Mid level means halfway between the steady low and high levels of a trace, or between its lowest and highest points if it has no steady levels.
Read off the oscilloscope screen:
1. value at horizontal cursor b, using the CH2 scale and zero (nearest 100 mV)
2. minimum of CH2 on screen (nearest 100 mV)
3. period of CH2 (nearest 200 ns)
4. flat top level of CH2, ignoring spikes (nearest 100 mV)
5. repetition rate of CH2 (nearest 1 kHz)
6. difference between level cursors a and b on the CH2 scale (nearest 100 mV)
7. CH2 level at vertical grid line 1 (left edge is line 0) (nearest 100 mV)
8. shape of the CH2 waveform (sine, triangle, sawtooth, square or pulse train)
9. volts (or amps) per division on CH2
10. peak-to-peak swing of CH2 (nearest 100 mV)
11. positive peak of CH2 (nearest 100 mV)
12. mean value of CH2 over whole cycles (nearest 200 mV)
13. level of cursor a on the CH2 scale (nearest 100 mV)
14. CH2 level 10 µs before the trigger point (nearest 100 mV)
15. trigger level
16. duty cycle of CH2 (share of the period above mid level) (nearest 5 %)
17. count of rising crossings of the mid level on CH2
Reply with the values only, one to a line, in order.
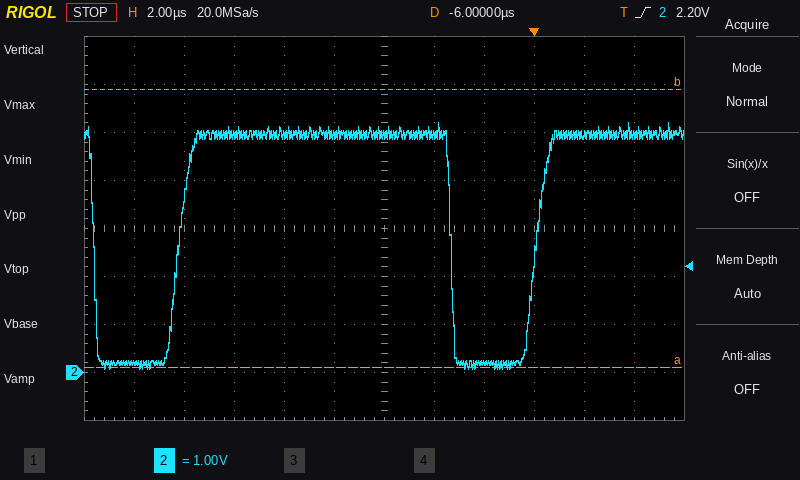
5.9 V
100 mV
14.2 µs
5.0 V
70 kHz
5.8 V
200 mV
pulse train
1 V
5.1 V
5.2 V
3.8 V
100 mV
5.0 V
2.20 V
75 %
2
